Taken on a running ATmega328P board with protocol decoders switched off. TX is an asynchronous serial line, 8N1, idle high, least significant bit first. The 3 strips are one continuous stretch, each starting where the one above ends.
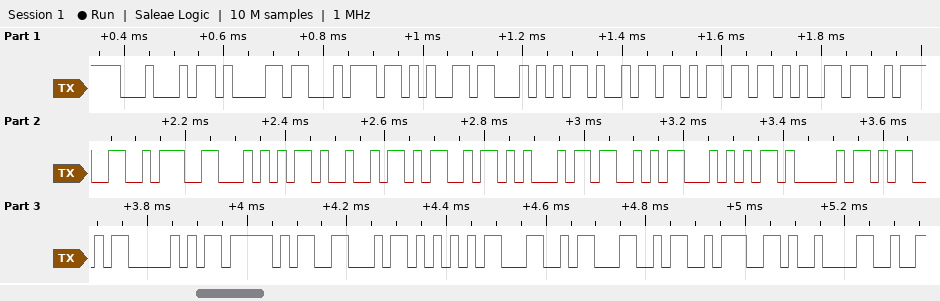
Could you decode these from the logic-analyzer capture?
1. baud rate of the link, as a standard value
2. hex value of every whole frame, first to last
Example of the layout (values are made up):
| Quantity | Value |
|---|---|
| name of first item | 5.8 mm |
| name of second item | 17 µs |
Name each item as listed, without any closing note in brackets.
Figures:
| Quantity | Value |
|---|---|
| baud rate of the link, as a standard value | 57600 baud |
| hex value of every whole frame, first to last | 0x44 0x61 0x74 0x65 0x54 0x69 0x6D 0x65 0x3A 0x3A 0x54 0x49 0x4D 0x45 0x53 0x54 0x41 0x4D 0x50 0x5F 0x46 0x55 0x4C 0x4C 0x3A 0x09 |
